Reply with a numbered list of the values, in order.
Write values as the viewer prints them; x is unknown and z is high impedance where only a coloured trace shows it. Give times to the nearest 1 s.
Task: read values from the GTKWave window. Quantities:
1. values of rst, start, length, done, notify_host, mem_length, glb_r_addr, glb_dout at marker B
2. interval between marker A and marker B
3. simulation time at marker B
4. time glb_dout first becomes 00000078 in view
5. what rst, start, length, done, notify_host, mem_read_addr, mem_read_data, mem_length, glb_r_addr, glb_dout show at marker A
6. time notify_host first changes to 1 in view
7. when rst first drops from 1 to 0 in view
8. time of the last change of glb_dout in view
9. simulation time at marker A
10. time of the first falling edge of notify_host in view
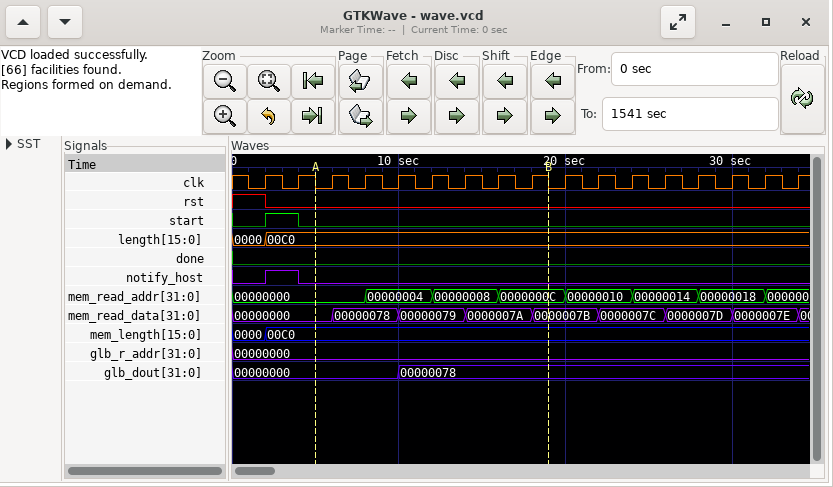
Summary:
1. rst=0, start=0, length=00C0, done=0, notify_host=0, mem_length=00C0, glb_r_addr=00000000, glb_dout=00000078
2. 14 s
3. 19 s
4. 10 s
5. rst=0, start=0, length=00C0, done=0, notify_host=0, mem_read_addr=00000000, mem_read_data=00000000, mem_length=00C0, glb_r_addr=00000000, glb_dout=00000000
6. 2 s
7. 2 s
8. 10 s
9. 5 s
10. 4 s
